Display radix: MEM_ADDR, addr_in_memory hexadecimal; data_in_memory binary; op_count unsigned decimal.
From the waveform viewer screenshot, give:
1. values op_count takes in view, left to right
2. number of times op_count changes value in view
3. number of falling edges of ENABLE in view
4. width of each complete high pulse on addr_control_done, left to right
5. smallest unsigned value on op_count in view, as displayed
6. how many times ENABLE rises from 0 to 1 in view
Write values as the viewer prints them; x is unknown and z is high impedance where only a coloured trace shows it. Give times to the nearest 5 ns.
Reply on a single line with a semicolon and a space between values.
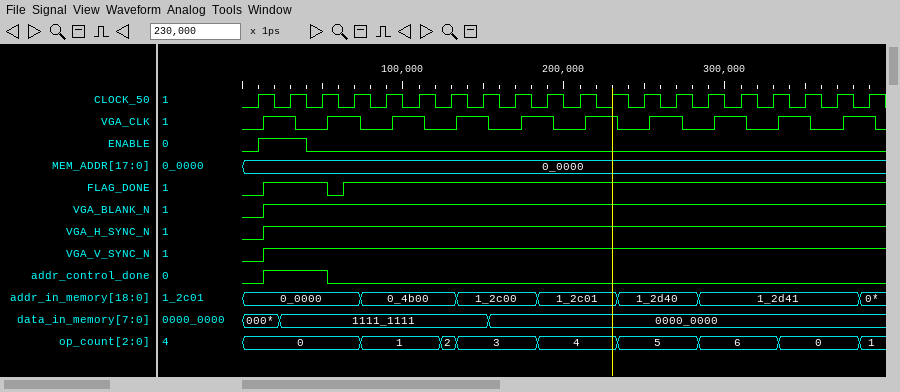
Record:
0, 1, 2, 3, 4, 5, 6, 0, 1; 8; 1; 40 ns; 0; 1
